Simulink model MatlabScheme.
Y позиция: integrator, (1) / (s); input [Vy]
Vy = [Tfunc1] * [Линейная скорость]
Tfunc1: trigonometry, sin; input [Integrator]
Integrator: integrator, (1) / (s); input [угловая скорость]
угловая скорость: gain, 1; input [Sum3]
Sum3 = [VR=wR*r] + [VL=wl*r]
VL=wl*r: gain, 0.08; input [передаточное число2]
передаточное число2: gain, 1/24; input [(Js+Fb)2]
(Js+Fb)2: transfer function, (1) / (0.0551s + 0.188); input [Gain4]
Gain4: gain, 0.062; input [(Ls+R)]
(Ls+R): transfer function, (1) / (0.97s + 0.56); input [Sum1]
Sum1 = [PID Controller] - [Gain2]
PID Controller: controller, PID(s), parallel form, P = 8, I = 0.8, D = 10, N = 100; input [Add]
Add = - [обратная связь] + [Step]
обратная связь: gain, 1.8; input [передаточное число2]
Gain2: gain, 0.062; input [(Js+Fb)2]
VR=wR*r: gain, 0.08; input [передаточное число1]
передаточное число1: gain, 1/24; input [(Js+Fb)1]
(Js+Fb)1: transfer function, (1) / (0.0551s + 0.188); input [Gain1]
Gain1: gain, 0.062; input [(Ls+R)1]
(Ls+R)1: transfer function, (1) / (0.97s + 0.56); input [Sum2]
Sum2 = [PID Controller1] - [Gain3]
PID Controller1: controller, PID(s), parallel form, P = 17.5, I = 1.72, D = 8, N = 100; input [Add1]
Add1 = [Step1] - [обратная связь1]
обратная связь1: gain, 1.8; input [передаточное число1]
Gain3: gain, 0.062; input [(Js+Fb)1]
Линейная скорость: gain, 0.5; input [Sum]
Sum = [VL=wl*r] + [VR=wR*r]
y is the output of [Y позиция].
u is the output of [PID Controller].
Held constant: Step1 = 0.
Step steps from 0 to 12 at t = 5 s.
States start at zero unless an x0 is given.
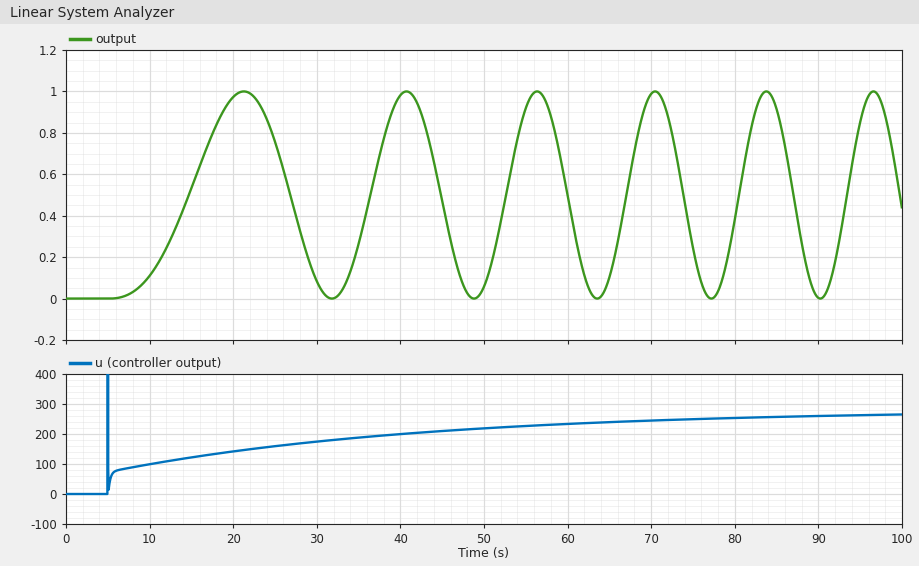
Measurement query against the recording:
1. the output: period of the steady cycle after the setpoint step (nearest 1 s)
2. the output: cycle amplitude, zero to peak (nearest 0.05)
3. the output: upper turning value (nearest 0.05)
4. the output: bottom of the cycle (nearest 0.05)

14 s
0.50
1.00
0.00
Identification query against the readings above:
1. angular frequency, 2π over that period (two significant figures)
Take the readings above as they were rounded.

0.45 rad/s
